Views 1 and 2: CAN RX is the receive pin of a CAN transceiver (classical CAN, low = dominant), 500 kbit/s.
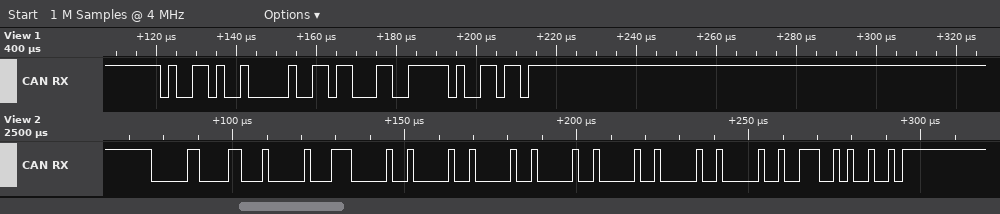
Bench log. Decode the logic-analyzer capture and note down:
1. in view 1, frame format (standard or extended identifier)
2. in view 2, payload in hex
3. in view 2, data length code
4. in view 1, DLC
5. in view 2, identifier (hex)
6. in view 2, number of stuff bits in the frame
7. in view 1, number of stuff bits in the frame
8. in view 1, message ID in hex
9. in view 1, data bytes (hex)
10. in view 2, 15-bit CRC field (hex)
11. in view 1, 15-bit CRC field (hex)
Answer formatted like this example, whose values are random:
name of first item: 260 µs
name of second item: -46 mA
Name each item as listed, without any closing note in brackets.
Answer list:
in view 1, frame format: standard
in view 2, payload in hex: 07 01 01 01 01 01 01 01
in view 2, data length code: 8
in view 1, DLC: 1
in view 2, identifier: 0x043
in view 2, number of stuff bits in the frame: 9
in view 1, number of stuff bits in the frame: 2
in view 1, message ID in hex: 0x4D2
in view 1, data bytes: B1
in view 2, 15-bit CRC field: 0x1CA4
in view 1, 15-bit CRC field: 0x4FCD
